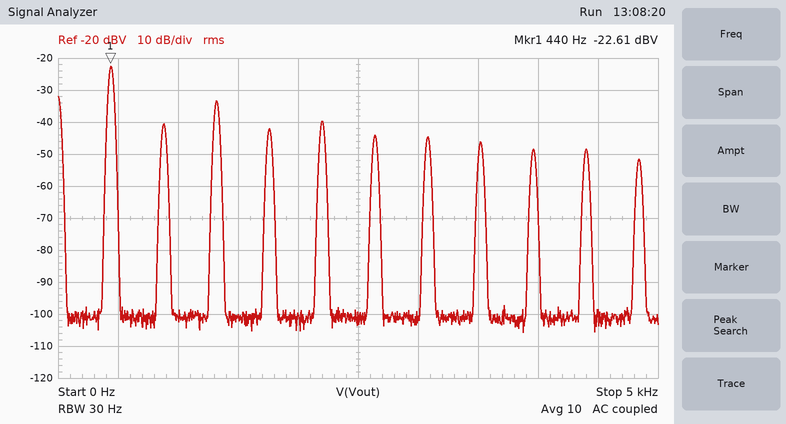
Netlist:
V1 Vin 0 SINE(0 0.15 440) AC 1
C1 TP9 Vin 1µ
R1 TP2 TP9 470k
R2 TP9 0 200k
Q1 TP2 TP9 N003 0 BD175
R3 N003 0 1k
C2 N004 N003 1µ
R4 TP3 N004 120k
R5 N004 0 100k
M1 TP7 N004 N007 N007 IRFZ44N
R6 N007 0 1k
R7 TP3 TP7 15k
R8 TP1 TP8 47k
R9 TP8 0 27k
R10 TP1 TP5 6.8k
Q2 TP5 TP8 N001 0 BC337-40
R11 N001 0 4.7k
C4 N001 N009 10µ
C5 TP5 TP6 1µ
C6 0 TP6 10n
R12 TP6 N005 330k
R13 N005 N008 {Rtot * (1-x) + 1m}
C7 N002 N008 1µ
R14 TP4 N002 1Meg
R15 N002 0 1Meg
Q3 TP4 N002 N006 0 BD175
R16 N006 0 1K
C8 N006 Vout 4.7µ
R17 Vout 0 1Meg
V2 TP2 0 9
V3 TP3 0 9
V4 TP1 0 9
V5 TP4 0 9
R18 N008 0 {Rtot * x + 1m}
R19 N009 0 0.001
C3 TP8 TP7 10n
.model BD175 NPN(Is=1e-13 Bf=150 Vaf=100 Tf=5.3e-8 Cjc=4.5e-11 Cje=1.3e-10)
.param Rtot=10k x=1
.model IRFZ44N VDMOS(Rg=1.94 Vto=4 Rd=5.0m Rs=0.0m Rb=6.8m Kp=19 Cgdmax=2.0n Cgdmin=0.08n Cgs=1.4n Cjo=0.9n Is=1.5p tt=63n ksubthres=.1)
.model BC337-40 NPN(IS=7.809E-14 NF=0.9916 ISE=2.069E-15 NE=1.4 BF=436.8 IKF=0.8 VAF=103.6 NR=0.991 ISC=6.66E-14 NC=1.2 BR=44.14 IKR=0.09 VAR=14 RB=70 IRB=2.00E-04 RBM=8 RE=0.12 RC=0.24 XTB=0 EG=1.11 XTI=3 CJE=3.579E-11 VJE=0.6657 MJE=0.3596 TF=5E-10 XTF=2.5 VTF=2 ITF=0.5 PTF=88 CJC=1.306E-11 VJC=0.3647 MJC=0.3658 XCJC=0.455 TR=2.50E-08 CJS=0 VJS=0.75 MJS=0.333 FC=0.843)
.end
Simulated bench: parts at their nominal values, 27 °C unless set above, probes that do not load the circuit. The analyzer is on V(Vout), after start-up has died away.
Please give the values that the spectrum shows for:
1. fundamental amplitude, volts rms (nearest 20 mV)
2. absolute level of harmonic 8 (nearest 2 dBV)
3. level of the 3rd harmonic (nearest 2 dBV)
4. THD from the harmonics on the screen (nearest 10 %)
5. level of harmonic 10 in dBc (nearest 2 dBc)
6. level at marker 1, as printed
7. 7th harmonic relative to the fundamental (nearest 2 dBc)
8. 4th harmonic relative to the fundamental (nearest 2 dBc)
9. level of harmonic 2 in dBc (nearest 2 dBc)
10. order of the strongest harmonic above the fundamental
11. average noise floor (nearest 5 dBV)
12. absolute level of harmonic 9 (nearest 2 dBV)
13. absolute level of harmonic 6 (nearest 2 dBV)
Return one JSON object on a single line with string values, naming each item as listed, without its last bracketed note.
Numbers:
{"fundamental amplitude, volts rms": "80 mV", "absolute level of harmonic 8": "-46 dBV", "level of the 3rd harmonic": "-34 dBV", "THD from the harmonics on the screen": "40 %", "level of harmonic 10 in dBc": "-26 dBc", "level at marker 1, as printed": "-22.61 dBV", "7th harmonic relative to the fundamental": "-22 dBc", "4th harmonic relative to the fundamental": "-20 dBc", "level of harmonic 2 in dBc": "-18 dBc", "order of the strongest harmonic above the fundamental": "3", "average noise floor": "-100 dBV", "absolute level of harmonic 9": "-48 dBV", "absolute level of harmonic 6": "-44 dBV"}
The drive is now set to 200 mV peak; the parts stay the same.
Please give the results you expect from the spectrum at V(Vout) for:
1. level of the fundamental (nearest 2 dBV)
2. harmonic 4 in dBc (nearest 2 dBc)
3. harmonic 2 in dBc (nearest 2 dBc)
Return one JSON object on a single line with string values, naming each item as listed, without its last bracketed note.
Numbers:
{"level of the fundamental": "-22 dBV", "harmonic 4 in dBc": "-22 dBc", "harmonic 2 in dBc": "-20 dBc"}
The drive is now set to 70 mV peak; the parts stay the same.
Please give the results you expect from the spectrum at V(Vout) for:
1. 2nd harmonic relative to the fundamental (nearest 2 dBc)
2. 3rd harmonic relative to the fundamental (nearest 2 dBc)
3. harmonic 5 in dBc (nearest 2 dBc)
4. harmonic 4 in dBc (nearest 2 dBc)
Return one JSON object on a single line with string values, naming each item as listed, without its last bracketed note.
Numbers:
{"2nd harmonic relative to the fundamental": "-14 dBc", "3rd harmonic relative to the fundamental": "-12 dBc", "harmonic 5 in dBc": "-22 dBc", "harmonic 4 in dBc": "-16 dBc"}
